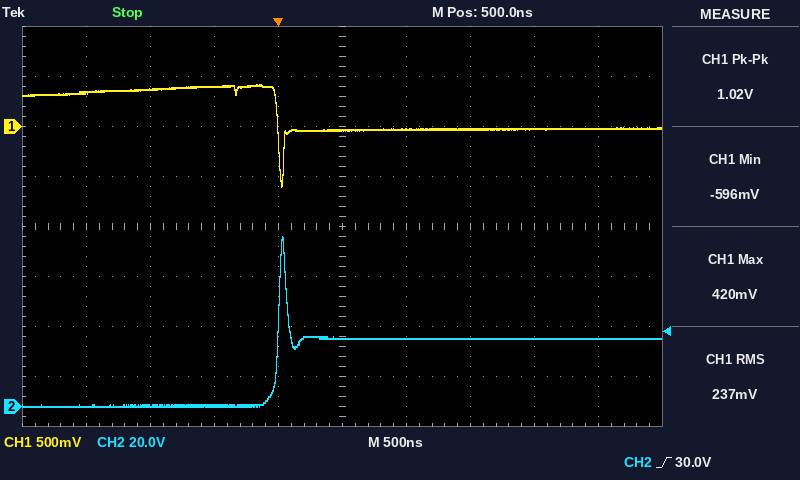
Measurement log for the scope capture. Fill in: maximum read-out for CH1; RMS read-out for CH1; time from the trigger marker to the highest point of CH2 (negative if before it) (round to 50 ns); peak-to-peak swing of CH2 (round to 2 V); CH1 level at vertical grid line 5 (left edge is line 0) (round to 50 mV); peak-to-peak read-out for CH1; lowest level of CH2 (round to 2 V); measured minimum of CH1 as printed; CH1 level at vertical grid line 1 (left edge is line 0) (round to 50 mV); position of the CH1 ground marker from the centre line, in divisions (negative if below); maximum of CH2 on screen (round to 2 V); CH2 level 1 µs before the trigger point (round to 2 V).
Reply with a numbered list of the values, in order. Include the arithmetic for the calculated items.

1. 420 mV
2. 237 mV
3. +50 ns
4. 68 V − (0 V) = 68 V
5. -50 mV
6. 1.02 V
7. 0 V
8. -596 mV
9. 350 mV
10. +2.0 div
11. 68 V
12. 0 V
